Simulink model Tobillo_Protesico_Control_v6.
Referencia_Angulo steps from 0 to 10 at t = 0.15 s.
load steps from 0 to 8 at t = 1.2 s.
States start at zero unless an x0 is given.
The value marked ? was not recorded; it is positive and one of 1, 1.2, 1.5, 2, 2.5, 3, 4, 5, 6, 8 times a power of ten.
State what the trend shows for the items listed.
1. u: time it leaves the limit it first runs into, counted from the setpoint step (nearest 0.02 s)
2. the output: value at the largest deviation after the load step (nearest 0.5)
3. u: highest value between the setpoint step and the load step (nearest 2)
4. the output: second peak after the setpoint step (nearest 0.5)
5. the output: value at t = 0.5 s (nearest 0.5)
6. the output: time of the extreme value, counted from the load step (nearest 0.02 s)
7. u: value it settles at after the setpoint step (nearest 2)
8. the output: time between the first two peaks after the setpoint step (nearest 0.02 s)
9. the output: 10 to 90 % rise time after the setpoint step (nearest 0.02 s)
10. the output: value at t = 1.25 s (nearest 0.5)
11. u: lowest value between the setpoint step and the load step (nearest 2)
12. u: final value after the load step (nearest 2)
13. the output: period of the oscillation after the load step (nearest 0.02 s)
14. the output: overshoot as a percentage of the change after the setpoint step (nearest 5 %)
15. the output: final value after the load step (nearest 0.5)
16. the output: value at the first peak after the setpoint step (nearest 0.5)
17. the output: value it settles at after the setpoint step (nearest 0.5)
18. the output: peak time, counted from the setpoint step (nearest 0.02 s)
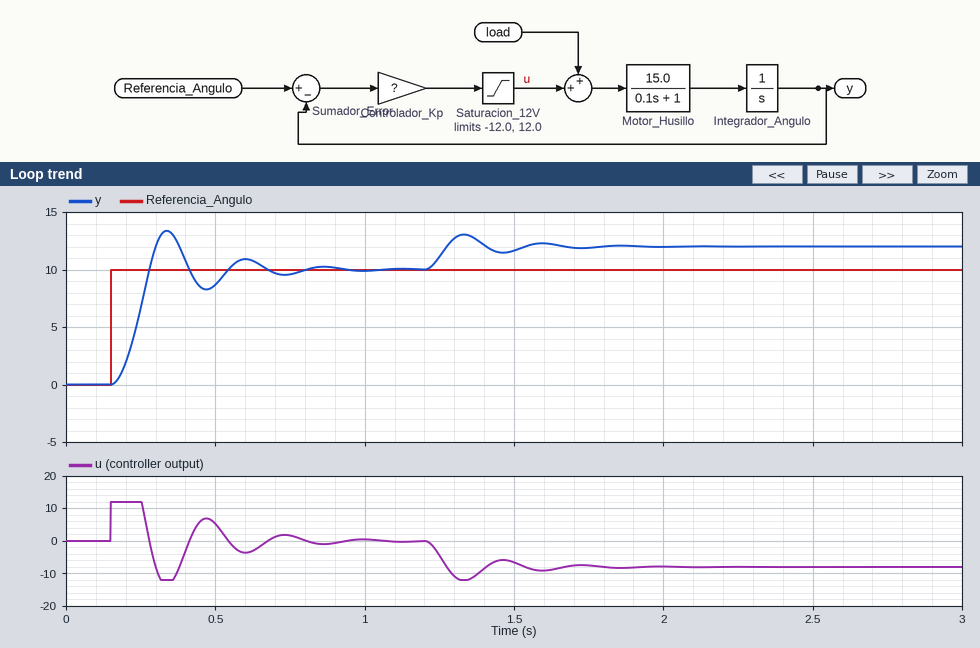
0.10 s
13.0
12
11.0
8.5
0.14 s
0
0.26 s
0.08 s
11.0
-12
-8
0.26 s
35 %
12.0
13.5
10.0
0.18 s
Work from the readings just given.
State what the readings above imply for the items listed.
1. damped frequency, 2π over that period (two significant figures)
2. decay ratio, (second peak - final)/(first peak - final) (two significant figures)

24 rad/s
0.29
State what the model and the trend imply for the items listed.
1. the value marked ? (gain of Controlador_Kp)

4
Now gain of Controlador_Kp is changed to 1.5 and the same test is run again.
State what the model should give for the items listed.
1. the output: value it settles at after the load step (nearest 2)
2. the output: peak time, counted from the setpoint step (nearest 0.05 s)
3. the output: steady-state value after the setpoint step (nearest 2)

16
0.25 s
10
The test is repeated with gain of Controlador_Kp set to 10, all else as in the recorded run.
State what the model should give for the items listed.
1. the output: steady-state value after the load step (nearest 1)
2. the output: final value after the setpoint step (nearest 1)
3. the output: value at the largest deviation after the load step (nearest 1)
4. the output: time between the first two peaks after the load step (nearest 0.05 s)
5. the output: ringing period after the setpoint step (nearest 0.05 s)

11
10
11
0.15 s
0.20 s
